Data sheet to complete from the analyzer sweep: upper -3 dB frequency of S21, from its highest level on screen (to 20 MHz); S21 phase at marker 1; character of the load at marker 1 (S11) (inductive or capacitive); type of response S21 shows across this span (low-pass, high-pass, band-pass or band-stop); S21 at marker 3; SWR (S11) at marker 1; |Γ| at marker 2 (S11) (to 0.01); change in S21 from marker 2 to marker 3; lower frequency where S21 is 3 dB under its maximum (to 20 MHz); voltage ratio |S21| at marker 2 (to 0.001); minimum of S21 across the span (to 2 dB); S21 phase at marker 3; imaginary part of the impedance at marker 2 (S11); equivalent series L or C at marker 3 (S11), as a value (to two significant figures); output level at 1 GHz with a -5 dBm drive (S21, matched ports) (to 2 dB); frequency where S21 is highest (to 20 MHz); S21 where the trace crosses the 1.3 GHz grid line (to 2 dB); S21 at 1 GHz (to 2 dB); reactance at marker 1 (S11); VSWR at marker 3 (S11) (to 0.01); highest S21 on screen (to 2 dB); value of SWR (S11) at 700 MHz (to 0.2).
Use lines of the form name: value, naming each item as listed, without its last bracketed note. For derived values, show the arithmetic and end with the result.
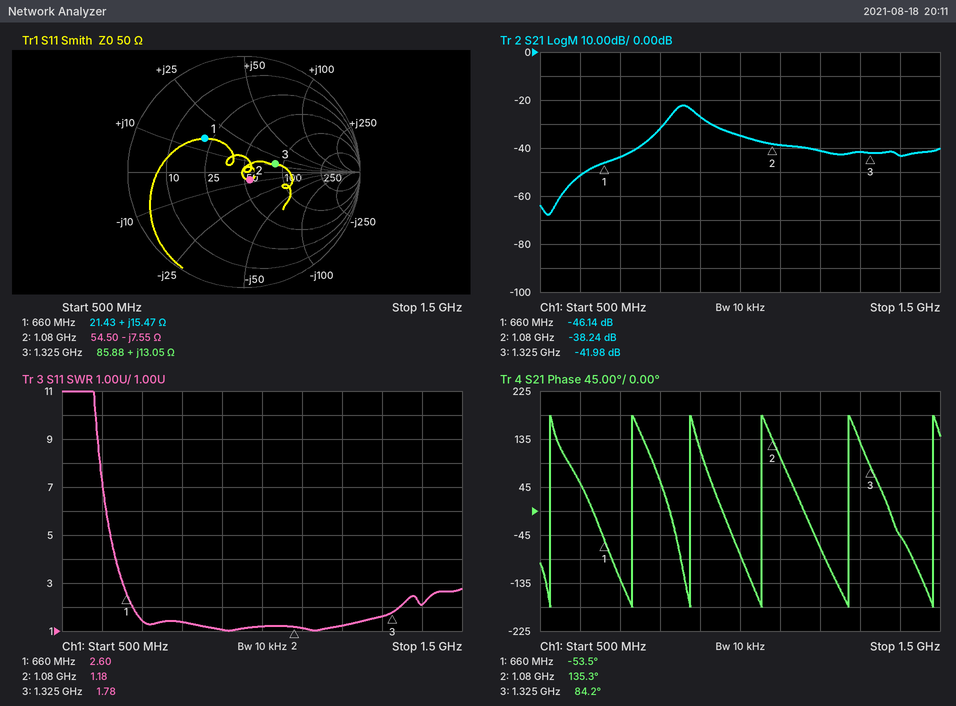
upper -3 dB frequency of S21, from its highest level on screen: 880 MHz
S21 phase at marker 1: -53.5°
character of the load at marker 1 (S11): inductive
type of response S21 shows across this span: band-pass
S21 at marker 3: -41.98 dB
SWR (S11) at marker 1: 2.60
|Γ| at marker 2 (S11): 0.08
change in S21 from marker 2 to marker 3: -41.98 − (-38.24) = -3.74 dB
lower frequency where S21 is 3 dB under its maximum: 840 MHz
voltage ratio |S21| at marker 2: 10^(-38.24/20) ≈ 0.012
minimum of S21 across the span: -68 dB
S21 phase at marker 3: 84.2°
imaginary part of the impedance at marker 2: -7.55 Ω
equivalent series L or C at marker 3 (S11), as a value: L = 13.05 Ω/(2π × 1.325 GHz) ≈ 1.6 nH
output level at 1 GHz with a -5 dBm drive (S21, matched ports): -5 dBm + (-34 dB) = -40 dBm
frequency where S21 is highest: 860 MHz
S21 where the trace crosses the 1.3 GHz grid line: -42 dB
S21 at 1 GHz: -34 dB
reactance at marker 1: +15.47 Ω
VSWR at marker 3 (S11): 1.78
highest S21 on screen: -22 dB
value of SWR (S11) at 700 MHz: 1.4
